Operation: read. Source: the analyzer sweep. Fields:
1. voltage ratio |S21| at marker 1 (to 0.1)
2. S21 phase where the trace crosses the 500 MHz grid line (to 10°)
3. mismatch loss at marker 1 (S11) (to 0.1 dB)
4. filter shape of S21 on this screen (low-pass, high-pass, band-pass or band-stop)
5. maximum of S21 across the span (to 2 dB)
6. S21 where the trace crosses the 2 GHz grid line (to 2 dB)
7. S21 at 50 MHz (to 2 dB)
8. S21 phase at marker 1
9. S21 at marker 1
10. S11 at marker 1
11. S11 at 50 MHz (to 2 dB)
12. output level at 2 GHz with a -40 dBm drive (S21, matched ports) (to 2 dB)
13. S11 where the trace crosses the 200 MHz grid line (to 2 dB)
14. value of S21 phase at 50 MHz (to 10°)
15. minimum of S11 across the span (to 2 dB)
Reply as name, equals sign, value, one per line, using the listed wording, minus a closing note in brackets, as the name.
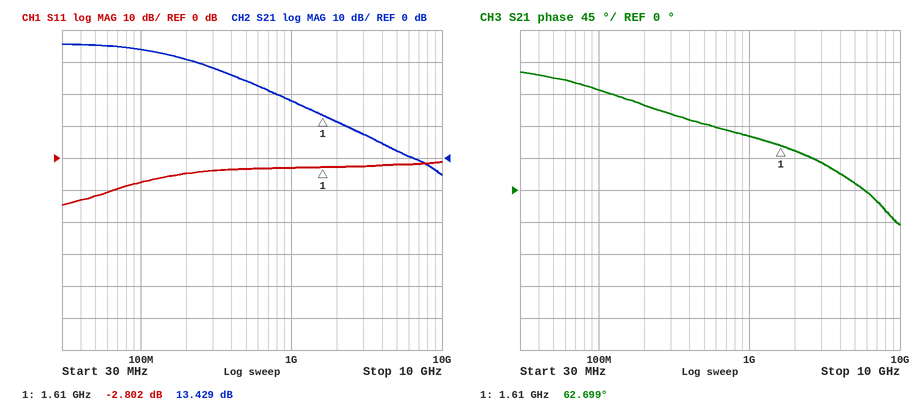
voltage ratio |S21| at marker 1 = 4.7
S21 phase where the trace crosses the 500 MHz grid line = 90°
mismatch loss at marker 1 (S11) = 3.2 dB
filter shape of S21 on this screen = low-pass
maximum of S21 across the span = 36 dB
S21 where the trace crosses the 2 GHz grid line = 12 dB
S21 at 50 MHz = 36 dB
S21 phase at marker 1 = 62.699°
S21 at marker 1 = 13.429 dB
S11 at marker 1 = -2.802 dB
S11 at 50 MHz = -12 dB
output level at 2 GHz with a -40 dBm drive (S21, matched ports) = -28 dBm
S11 where the trace crosses the 200 MHz grid line = -4 dB
value of S21 phase at 50 MHz = 160°
minimum of S11 across the span = -14 dB
